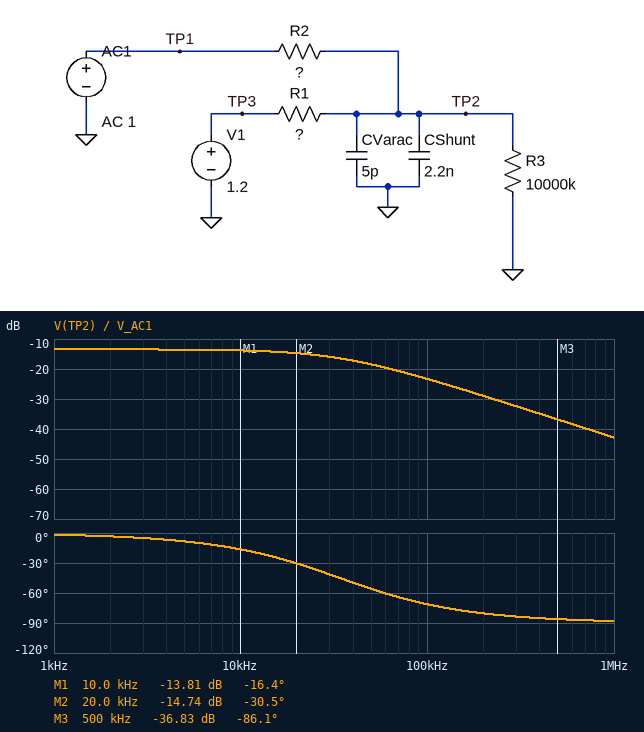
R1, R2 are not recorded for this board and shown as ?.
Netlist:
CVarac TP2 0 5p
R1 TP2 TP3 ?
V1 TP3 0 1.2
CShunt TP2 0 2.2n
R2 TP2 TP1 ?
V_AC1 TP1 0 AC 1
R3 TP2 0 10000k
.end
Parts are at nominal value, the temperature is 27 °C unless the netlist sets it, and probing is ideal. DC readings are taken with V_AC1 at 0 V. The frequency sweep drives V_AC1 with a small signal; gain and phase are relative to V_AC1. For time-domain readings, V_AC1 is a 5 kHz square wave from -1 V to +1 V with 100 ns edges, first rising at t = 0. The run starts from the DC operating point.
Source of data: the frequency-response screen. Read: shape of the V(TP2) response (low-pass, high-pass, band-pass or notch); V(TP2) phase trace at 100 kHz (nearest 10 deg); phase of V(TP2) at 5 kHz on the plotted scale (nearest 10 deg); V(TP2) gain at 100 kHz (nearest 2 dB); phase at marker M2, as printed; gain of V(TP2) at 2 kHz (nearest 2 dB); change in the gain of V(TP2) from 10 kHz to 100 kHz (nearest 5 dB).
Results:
low-pass
-70 deg
-10 deg
-24 dB
-30.5 deg
-14 dB
-10 dB
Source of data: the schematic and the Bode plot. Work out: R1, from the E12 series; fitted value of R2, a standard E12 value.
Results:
2.7 kΩ
10 kΩ
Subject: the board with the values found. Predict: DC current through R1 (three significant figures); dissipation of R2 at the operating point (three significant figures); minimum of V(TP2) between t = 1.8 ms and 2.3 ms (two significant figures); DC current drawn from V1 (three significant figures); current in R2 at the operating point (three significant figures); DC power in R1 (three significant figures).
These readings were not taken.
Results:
94.6 µA
89.2 µW
730 mV
94.6 µA
94.5 µA
24.1 µW
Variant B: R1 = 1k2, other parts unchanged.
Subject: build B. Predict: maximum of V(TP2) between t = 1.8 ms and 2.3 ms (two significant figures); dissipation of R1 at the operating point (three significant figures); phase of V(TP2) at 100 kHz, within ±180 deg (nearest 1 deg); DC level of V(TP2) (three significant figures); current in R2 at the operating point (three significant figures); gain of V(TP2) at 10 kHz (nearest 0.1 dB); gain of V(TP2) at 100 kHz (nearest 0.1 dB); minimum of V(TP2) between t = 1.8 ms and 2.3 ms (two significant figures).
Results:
1.2 V
13.8 µW
-56 deg
1.07 V
107 µA
-19.5 dB
-24.5 dB
960 mV
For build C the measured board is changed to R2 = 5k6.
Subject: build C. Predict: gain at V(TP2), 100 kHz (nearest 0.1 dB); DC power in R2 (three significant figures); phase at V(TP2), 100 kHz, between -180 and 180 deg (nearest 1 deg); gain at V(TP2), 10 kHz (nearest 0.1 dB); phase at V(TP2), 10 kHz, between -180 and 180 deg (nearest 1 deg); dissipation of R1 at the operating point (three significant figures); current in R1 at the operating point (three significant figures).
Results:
-18.4 dB
117 µW
-68 deg
-10.0 dB
-14 deg
56.5 µW
145 µA
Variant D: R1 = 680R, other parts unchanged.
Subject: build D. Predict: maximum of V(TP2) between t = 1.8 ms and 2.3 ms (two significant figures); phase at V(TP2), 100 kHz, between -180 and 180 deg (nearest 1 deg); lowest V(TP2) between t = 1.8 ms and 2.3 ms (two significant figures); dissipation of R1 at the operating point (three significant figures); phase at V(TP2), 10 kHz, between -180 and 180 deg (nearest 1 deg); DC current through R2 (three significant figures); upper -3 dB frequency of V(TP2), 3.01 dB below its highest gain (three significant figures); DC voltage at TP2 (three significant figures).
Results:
1.2 V
-41 deg
1.1 V
8.60 µW
-5 deg
112 µA
113 kHz
1.12 V
